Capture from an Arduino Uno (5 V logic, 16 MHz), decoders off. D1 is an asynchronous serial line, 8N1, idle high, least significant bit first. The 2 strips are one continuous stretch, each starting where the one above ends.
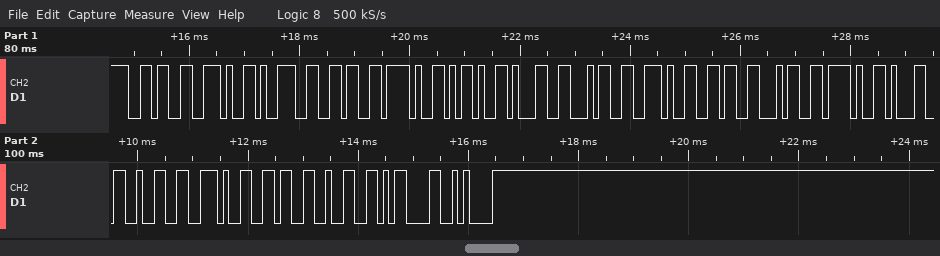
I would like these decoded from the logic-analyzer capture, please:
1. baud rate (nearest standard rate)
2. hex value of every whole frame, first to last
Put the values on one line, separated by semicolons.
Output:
9600 baud; 36 2E 39 36 2F 2D 31 34 2E 36 34 2F 31 32 2E 36 32 0D 0A
